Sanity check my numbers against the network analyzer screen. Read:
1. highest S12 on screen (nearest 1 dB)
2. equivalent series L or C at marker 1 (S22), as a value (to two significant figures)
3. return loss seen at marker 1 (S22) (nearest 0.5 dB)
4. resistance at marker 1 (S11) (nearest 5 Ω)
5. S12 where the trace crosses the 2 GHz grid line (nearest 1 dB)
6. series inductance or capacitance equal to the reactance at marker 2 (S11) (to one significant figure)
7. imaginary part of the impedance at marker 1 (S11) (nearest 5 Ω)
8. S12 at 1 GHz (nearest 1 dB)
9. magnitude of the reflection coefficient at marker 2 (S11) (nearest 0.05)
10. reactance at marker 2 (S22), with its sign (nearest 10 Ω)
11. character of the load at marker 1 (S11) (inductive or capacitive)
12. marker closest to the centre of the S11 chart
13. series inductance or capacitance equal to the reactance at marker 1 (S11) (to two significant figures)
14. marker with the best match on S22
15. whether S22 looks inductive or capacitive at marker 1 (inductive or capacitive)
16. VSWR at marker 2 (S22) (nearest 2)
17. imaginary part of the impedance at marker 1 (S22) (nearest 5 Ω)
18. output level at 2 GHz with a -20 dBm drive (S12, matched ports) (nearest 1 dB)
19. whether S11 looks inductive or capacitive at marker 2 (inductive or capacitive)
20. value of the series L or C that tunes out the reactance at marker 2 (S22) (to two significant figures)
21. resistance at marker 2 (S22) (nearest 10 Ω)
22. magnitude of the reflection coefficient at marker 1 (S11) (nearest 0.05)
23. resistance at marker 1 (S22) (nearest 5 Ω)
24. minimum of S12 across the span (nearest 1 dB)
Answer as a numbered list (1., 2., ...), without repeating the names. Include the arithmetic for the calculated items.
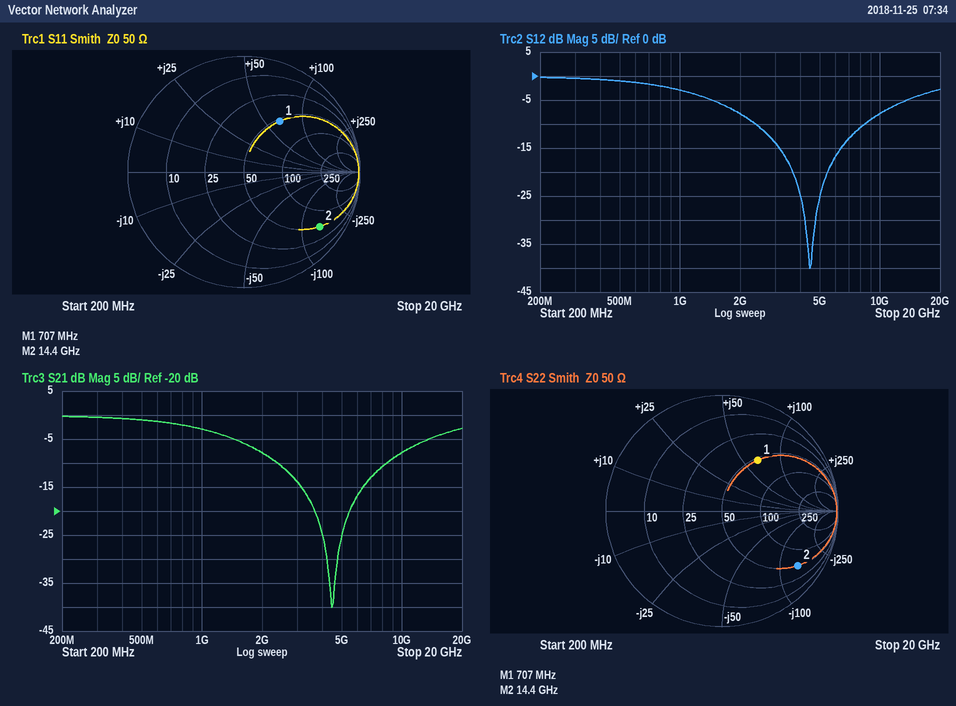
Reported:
1. 0 dB
2. L = 65 Ω/(2π × 707 MHz) ≈ 15 nH
3. 5.5 dB
4. 55 Ω
5. -8 dB
6. C = 1/(2π × 14.4 GHz × 140 Ω) ≈ 78.9 fF, so 80 fF to one significant figure
7. +65 Ω
8. -3 dB
9. 0.80
10. -140 Ω
11. inductive
12. marker 1
13. L = 65 Ω/(2π × 707 MHz) ≈ 15 nH
14. marker 1
15. inductive
16. 10
17. +65 Ω
18. -20 dBm + (-8 dB) = -28 dBm
19. capacitive
20. L = 140 Ω/(2π × 14.4 GHz) ≈ 1.5 nH
21. 50 Ω
22. 0.55
23. 55 Ω
24. -40 dB
